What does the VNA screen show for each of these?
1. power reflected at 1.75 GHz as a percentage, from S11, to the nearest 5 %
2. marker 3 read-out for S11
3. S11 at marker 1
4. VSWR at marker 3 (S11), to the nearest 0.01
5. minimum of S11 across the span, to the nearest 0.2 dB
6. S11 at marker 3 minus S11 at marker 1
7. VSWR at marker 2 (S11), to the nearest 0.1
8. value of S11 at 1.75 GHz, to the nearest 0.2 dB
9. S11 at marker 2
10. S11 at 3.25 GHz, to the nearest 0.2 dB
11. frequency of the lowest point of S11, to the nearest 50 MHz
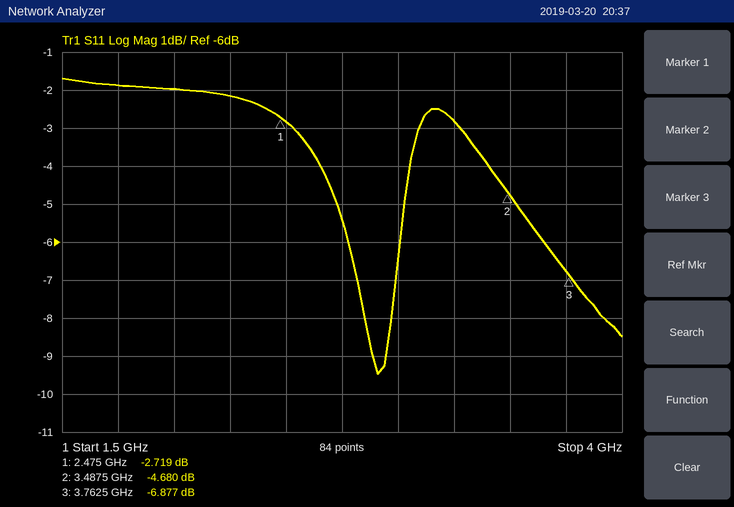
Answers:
65 %
-6.877 dB
-2.719 dB
2.66
-9.4 dB
-4.158 dB
3.8
-1.8 dB
-4.680 dB
-2.8 dB
2.90 GHz
